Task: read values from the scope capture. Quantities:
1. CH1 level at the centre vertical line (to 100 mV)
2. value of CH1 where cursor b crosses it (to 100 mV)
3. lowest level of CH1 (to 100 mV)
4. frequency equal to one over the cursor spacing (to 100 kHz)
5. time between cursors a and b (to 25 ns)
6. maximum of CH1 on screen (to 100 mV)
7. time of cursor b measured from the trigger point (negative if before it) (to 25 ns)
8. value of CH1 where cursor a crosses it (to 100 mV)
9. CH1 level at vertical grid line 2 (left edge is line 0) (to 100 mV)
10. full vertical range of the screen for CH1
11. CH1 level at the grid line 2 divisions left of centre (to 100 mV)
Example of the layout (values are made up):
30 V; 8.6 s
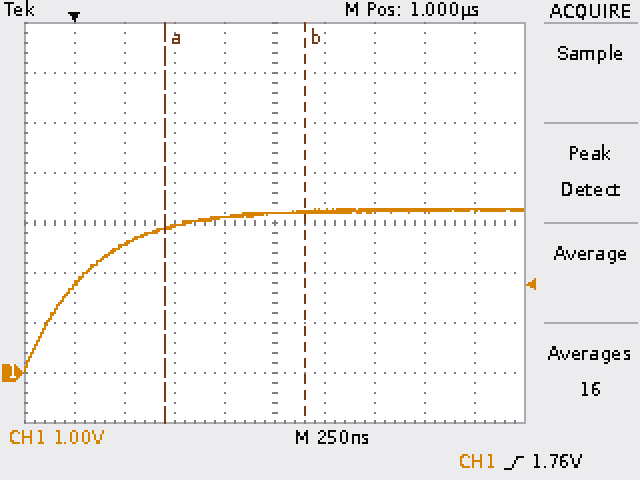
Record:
3.2 V; 3.2 V; 0.0 V; 1.4 MHz; 700 ns; 3.3 V; +1.150 µs; 2.9 V; 2.6 V; 8 V; 2.9 V
